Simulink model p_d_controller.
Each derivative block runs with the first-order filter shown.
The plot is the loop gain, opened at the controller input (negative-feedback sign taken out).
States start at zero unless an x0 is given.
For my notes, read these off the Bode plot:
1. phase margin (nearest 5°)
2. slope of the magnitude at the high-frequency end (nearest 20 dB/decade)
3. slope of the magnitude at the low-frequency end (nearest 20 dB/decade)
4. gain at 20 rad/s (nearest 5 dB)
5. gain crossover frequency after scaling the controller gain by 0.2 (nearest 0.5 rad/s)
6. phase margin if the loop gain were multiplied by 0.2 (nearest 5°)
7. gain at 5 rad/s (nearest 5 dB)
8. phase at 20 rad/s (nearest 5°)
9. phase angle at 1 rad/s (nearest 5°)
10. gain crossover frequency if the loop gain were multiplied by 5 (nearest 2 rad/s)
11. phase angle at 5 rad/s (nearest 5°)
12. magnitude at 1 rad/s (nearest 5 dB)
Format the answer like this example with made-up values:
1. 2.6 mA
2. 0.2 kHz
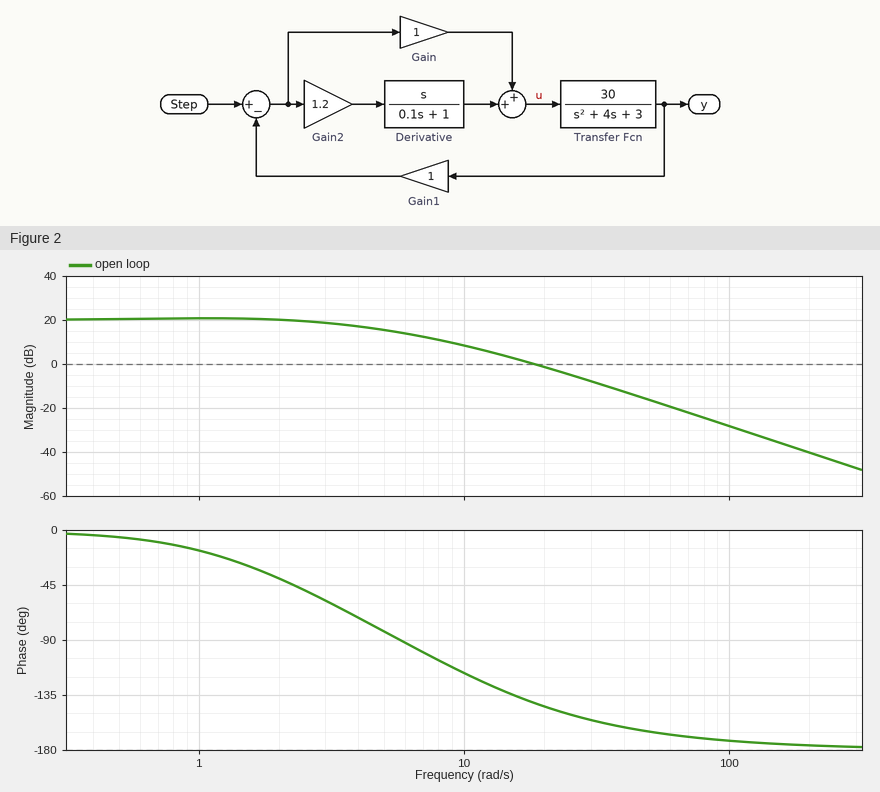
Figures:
1. 40°
2. -40 dB/decade
3. 0 dB/decade
4. 0 dB
5. 6.0 rad/s
6. 90°
7. 15 dB
8. -145°
9. -15°
10. 44 rad/s
11. -85°
12. 20 dB
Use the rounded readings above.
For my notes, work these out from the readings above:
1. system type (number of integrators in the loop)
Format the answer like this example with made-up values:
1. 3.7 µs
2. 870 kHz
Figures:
1. 0
